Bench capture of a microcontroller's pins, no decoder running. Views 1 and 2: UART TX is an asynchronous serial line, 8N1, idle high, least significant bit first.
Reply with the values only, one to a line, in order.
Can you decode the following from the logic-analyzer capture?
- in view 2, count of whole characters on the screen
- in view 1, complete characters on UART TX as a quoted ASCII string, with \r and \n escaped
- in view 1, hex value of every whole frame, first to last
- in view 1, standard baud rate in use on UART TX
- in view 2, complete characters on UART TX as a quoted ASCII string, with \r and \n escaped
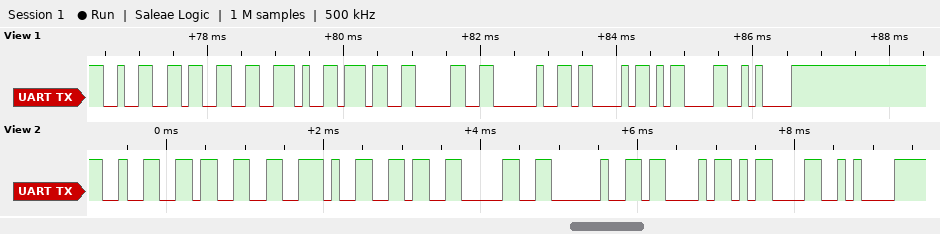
9
"23.70 C\r\n"
32 33 2E 37 30 20 43 0D 0A
9600 baud
"23.60 C\r\n"
